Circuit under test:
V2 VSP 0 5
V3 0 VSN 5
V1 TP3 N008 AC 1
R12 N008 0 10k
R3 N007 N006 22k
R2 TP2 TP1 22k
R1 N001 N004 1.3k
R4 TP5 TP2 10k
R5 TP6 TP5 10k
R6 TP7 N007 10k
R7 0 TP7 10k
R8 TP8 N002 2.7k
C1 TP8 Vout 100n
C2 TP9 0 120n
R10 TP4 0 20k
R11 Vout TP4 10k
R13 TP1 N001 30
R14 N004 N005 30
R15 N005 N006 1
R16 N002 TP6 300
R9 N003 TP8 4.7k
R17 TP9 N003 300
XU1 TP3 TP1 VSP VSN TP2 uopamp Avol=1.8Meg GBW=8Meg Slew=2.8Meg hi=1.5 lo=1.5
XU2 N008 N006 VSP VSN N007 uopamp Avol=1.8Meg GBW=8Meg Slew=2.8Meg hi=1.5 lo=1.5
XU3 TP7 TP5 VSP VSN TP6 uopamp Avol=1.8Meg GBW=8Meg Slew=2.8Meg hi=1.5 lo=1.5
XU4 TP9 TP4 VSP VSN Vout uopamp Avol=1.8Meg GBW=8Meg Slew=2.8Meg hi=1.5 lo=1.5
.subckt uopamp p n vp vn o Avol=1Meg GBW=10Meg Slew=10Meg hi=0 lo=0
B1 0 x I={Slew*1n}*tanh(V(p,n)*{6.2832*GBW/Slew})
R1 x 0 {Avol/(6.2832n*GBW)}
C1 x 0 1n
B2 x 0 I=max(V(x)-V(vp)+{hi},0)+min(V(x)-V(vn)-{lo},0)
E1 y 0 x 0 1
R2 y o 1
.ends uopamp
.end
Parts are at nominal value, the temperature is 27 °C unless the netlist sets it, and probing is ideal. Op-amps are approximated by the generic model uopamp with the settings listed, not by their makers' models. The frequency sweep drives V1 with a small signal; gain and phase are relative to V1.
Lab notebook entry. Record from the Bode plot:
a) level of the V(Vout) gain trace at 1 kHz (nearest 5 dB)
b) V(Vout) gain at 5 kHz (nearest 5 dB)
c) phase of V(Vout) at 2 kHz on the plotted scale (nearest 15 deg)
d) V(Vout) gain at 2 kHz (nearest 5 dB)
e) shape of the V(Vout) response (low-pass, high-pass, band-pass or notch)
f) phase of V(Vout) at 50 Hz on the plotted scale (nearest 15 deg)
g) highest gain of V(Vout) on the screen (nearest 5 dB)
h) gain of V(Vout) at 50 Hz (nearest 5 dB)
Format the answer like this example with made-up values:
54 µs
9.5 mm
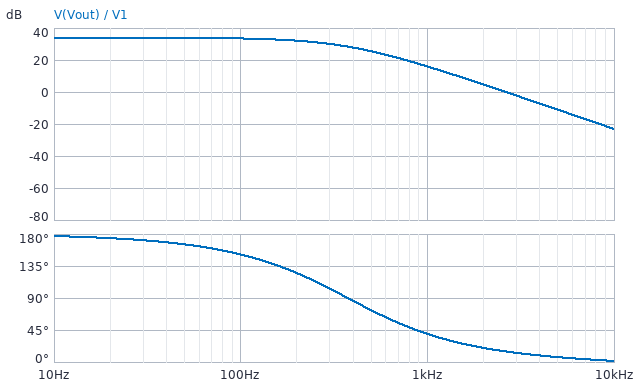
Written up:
15 dB
-10 dB
15 deg
5 dB
low-pass
165 deg
35 dB
35 dB
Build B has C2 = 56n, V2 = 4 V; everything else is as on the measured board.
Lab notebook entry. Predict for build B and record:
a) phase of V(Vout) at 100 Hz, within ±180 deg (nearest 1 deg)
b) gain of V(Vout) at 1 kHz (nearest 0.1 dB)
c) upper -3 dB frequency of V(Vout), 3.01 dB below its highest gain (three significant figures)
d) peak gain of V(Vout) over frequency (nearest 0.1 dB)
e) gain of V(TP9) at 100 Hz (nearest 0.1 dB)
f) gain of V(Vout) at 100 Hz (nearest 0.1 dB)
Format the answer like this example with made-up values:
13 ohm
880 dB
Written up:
169 deg
24.5 dB
639 Hz
35.1 dB
30.6 dB
34.1 dB
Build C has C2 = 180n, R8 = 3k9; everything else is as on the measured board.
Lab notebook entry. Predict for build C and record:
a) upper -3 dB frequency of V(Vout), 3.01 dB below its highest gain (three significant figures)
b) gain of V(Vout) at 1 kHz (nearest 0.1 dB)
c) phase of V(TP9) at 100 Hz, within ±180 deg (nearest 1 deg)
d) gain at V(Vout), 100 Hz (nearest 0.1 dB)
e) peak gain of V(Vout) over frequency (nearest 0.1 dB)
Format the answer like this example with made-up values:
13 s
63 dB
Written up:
133 Hz
9.6 dB
133 deg
32.1 dB
34.0 dB
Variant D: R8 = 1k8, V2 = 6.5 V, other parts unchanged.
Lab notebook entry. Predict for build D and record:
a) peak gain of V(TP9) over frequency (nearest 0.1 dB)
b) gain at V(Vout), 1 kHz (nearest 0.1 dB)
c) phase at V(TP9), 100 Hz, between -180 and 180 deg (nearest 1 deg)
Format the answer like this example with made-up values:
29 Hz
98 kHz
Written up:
30.5 dB
18.2 dB
154 deg
